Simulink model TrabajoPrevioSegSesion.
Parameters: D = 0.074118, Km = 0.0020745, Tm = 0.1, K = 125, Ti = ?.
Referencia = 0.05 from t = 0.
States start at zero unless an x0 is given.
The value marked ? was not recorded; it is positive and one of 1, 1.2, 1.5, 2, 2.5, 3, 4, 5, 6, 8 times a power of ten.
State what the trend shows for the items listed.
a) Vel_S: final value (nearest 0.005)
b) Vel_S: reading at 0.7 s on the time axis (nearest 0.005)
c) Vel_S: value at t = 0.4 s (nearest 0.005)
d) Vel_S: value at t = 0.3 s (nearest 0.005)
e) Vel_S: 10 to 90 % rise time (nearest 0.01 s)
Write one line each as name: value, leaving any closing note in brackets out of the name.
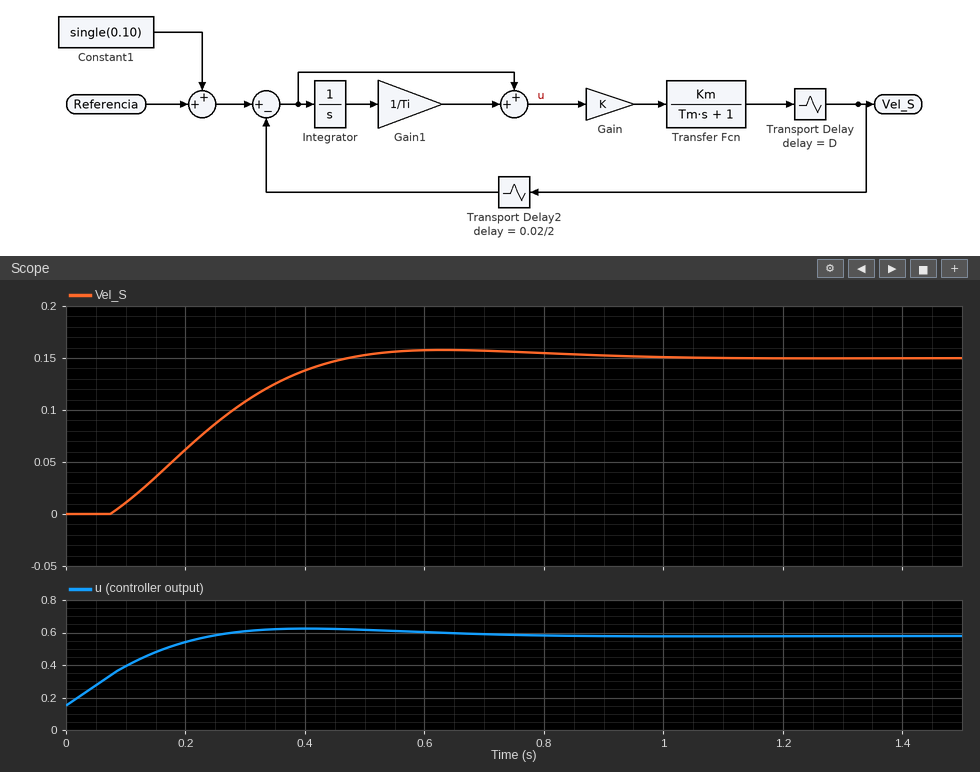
Vel_S: final value: 0.150
Vel_S: reading at 0.7 s on the time axis: 0.155
Vel_S: value at t = 0.4 s: 0.140
Vel_S: value at t = 0.3 s: 0.110
Vel_S: 10 to 90 % rise time: 0.28 s
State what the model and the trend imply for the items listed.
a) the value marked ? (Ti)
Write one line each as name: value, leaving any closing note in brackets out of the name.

the value marked ?: 0.06
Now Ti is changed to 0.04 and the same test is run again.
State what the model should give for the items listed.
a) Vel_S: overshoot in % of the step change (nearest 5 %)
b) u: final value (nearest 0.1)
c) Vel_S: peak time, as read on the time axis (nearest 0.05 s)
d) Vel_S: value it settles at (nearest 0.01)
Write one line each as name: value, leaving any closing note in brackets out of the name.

Vel_S: overshoot in % of the step change: 25 %
u: final value: 0.6
Vel_S: peak time, as read on the time axis: 0.45 s
Vel_S: value it settles at: 0.15
